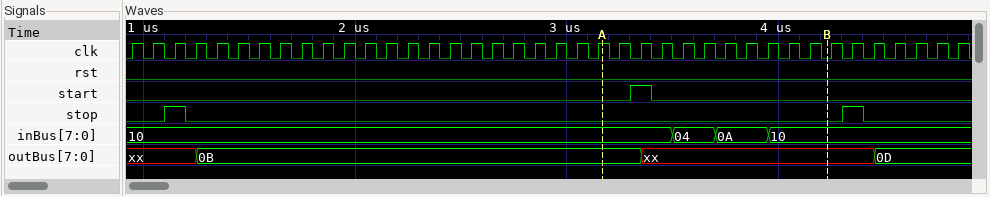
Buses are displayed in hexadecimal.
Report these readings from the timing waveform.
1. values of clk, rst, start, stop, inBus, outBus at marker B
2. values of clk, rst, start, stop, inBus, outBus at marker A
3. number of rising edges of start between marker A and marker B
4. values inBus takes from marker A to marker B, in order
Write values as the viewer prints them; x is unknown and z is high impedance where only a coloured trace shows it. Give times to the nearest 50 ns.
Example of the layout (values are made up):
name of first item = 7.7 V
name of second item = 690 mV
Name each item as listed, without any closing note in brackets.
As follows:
values of clk, rst, start, stop, inBus, outBus at marker B = clk=0, rst=0, start=0, stop=0, inBus=10, outBus=xx
values of clk, rst, start, stop, inBus, outBus at marker A = clk=1, rst=0, start=0, stop=0, inBus=10, outBus=0B
number of rising edges of start between marker A and marker B = 1
values inBus takes from marker A to marker B, in order = 10, 04, 0A, 10
